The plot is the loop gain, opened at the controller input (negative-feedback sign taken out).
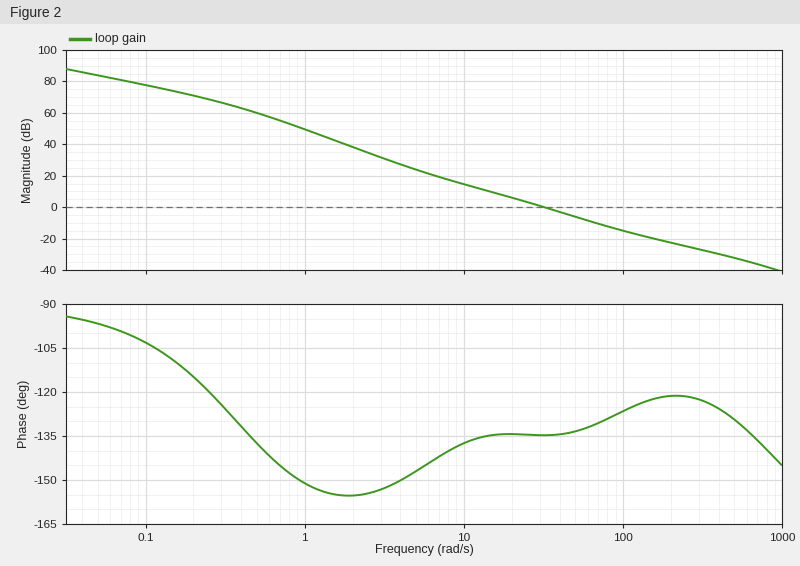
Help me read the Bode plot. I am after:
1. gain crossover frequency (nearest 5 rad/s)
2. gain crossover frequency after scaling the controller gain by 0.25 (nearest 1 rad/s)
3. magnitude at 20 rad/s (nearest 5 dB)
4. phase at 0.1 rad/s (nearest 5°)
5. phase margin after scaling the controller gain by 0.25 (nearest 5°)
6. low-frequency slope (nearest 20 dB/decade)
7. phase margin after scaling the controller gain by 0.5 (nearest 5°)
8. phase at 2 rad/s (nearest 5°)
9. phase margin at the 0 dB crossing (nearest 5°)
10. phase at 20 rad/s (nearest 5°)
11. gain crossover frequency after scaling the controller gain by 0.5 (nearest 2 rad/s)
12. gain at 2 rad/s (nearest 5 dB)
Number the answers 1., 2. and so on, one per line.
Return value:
1. 30 rad/s
2. 12 rad/s
3. 5 dB
4. -105°
5. 45°
6. -20 dB/decade
7. 45°
8. -155°
9. 45°
10. -135°
11. 20 rad/s
12. 40 dB
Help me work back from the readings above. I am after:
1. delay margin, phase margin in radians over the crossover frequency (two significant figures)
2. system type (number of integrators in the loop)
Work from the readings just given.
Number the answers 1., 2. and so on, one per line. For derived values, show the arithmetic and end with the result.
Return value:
1. 45 × π / 180 / 30 = 0.026 s
2. 1
